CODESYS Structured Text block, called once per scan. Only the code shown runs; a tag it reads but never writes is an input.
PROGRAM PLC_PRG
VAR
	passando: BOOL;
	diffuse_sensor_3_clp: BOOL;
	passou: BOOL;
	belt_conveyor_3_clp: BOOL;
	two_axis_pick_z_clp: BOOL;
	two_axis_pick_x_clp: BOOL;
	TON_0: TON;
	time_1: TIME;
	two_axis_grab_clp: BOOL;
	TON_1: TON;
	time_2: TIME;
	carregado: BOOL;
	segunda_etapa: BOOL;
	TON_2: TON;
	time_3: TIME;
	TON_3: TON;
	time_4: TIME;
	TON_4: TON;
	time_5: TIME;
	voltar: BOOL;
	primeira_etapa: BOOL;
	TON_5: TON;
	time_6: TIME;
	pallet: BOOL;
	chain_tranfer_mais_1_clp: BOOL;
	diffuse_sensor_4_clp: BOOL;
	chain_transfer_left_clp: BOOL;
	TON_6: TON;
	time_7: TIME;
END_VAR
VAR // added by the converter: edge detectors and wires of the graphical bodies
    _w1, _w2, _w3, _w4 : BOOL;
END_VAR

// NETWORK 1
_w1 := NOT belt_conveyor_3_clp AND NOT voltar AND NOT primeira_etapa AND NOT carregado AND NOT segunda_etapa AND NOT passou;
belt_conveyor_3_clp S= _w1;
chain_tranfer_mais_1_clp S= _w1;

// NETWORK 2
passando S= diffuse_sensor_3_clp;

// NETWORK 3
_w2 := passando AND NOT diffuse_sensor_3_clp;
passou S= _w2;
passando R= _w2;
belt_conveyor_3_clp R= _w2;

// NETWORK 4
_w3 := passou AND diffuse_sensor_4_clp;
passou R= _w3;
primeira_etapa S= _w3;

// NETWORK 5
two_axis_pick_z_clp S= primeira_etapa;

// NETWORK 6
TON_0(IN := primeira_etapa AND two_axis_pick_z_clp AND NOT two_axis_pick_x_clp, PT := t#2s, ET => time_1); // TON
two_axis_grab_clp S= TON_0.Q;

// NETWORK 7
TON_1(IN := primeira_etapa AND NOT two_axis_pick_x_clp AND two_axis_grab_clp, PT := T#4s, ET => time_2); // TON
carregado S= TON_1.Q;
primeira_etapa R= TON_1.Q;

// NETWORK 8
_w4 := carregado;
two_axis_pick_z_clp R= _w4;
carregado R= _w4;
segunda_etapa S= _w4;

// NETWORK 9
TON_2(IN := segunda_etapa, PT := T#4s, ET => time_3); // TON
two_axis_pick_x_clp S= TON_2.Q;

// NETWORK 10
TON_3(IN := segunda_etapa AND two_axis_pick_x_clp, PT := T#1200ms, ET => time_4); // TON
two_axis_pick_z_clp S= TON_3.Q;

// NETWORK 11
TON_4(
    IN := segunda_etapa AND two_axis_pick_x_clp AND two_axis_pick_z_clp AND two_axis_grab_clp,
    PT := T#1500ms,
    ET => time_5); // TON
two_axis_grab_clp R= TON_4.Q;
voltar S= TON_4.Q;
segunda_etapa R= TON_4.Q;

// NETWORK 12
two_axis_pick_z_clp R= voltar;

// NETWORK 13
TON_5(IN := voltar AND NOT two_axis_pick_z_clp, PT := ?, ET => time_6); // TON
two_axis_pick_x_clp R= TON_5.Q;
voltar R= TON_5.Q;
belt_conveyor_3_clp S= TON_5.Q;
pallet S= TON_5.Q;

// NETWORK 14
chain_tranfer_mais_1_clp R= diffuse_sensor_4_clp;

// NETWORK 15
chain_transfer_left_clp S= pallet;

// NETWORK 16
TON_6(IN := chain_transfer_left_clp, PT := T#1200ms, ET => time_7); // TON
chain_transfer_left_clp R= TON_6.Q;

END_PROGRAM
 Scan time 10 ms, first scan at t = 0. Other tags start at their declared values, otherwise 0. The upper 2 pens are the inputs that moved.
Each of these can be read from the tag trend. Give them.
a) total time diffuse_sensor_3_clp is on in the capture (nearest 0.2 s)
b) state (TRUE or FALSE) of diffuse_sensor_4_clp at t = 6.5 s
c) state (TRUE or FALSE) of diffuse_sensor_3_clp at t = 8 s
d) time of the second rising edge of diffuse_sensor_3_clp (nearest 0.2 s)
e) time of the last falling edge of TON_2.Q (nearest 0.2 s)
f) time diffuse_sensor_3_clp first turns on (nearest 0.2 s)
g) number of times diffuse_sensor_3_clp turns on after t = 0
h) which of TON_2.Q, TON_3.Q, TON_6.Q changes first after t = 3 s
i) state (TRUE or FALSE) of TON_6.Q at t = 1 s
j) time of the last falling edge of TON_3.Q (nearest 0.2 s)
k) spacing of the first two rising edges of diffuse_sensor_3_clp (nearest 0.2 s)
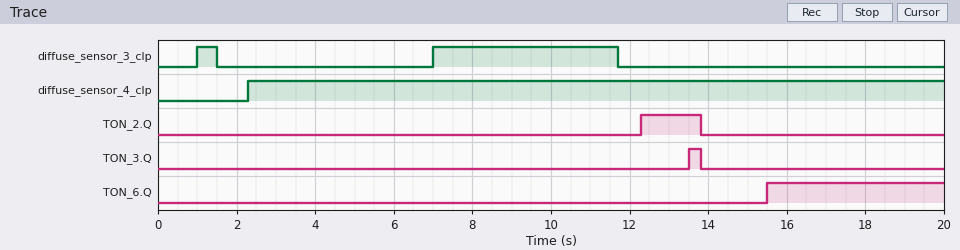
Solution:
5.2 s
TRUE
TRUE
7.0 s
13.8 s
1.0 s
2
TON_2.Q
FALSE
13.8 s
6.0 s
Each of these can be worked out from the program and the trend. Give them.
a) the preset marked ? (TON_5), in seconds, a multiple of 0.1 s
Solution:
0.5 s
